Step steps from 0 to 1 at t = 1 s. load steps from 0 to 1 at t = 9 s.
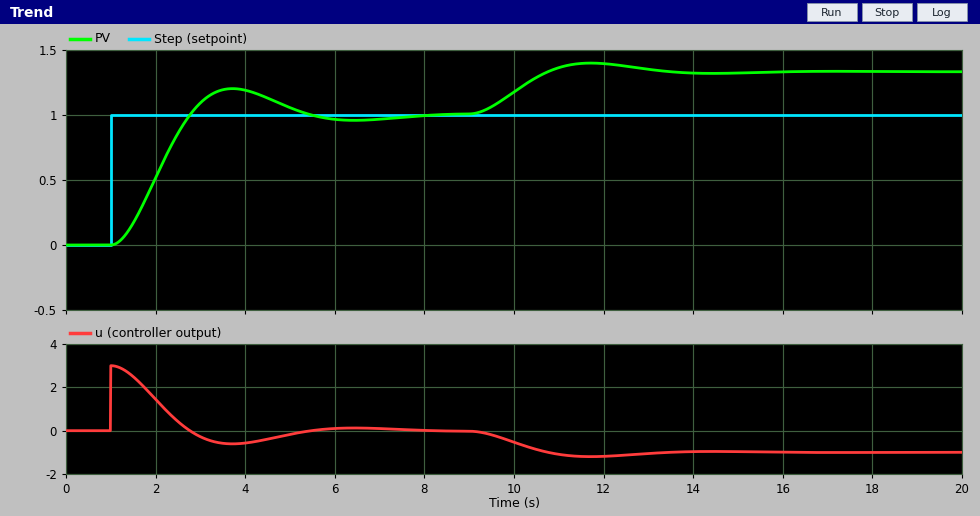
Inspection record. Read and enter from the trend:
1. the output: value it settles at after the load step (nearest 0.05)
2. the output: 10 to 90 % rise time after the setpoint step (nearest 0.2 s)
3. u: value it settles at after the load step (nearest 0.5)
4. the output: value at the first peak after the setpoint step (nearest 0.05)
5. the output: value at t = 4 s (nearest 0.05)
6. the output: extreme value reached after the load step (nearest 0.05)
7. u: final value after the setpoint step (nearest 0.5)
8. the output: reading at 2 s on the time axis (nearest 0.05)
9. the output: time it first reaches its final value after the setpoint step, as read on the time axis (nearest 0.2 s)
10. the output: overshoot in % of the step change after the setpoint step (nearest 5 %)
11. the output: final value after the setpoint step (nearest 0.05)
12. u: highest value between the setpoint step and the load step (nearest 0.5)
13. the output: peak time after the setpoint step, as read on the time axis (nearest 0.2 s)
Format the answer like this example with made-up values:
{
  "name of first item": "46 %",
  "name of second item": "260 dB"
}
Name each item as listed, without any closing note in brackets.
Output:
{
  "the output: value it settles at after the load step": "1.35",
  "the output: 10 to 90 % rise time after the setpoint step": "1.2 s",
  "u: value it settles at after the load step": "-1.0",
  "the output: value at the first peak after the setpoint step": "1.20",
  "the output: value at t = 4 s": "1.20",
  "the output: extreme value reached after the load step": "1.40",
  "u: final value after the setpoint step": "0.0",
  "the output: reading at 2 s on the time axis": "0.50",
  "the output: time it first reaches its final value after the setpoint step, as read on the time axis": "2.8 s",
  "the output: overshoot in % of the step change after the setpoint step": "20 %",
  "the output: final value after the setpoint step": "1.00",
  "u: highest value between the setpoint step and the load step": "3.0",
  "the output: peak time after the setpoint step, as read on the time axis": "3.8 s"
}
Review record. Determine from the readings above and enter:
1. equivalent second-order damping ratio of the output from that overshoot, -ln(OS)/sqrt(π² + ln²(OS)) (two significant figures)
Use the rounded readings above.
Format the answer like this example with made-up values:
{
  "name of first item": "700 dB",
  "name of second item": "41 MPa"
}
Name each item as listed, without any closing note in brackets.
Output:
{
  "equivalent second-order damping ratio of the output from that overshoot, -ln(OS)/sqrt(π² + ln²(OS))": "0.46"
}
